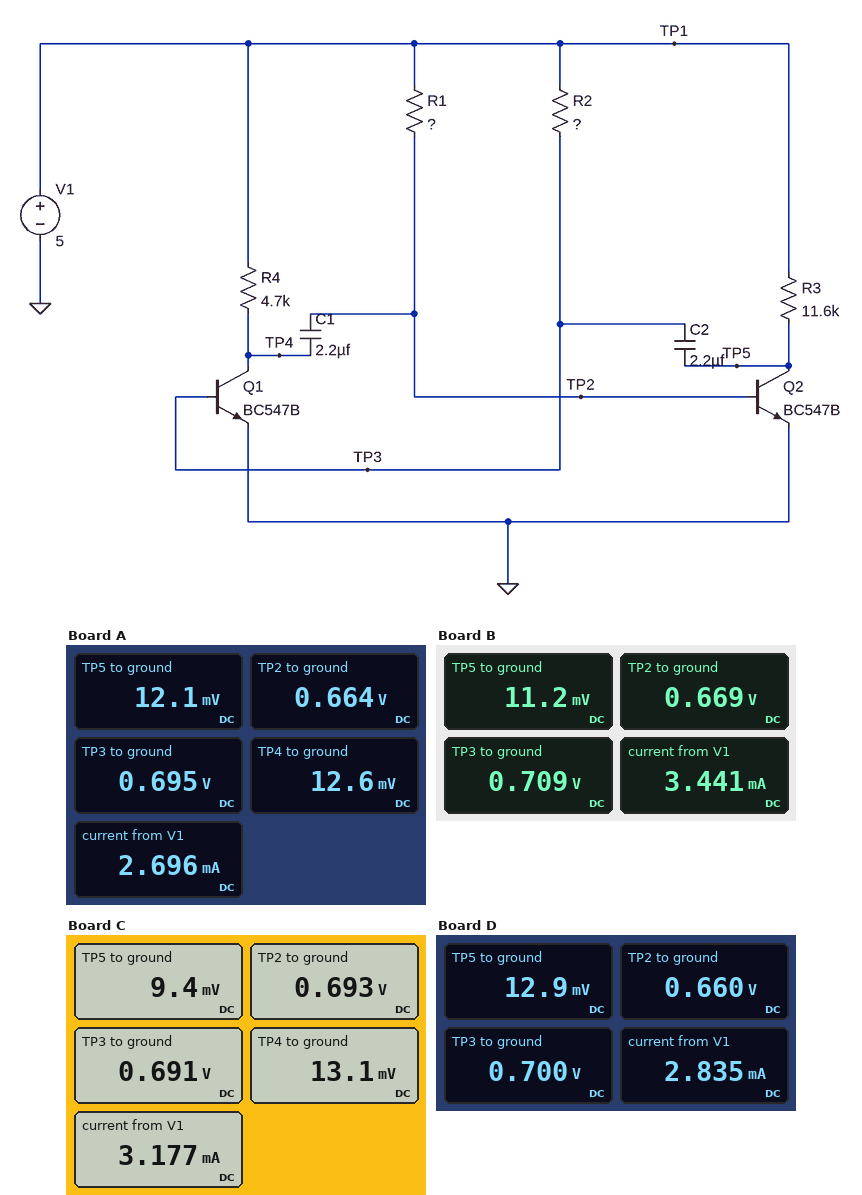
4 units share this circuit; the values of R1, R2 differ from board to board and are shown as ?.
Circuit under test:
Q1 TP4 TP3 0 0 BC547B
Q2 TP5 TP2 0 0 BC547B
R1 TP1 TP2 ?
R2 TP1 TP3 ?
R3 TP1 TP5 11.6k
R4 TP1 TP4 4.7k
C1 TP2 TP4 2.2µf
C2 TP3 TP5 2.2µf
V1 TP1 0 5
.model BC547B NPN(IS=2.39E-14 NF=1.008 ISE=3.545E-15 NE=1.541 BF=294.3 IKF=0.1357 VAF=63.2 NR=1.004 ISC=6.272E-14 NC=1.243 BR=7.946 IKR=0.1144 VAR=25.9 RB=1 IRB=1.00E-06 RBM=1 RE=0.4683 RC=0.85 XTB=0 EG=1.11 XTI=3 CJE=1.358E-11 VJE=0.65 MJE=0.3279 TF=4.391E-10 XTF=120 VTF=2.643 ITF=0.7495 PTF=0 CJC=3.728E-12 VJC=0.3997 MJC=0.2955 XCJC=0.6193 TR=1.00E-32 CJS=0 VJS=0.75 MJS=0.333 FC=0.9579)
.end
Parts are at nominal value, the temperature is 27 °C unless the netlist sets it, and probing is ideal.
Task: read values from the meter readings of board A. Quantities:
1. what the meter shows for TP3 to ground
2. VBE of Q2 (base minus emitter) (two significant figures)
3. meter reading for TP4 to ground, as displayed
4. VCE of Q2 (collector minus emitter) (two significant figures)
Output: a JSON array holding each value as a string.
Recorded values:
["0.695 V", "660 mV", "12.6 mV", "12 mV"]
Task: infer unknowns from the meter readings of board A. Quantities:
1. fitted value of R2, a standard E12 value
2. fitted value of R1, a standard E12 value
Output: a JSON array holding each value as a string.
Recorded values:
["4.7 kΩ", "15 kΩ"]
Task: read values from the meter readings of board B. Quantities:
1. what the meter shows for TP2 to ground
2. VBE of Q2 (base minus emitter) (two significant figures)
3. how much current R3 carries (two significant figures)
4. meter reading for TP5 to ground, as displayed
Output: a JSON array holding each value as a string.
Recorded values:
["0.669 V", "670 mV", "430 µA", "11.2 mV"]
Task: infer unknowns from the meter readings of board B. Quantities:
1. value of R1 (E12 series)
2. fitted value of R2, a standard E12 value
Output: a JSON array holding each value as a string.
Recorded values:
["12 kΩ", "2.7 kΩ"]
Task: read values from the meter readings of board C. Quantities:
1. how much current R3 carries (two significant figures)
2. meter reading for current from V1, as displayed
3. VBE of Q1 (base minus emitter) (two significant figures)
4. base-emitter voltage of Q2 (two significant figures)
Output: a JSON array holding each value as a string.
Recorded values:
["430 µA", "3.177 mA", "690 mV", "690 mV"]
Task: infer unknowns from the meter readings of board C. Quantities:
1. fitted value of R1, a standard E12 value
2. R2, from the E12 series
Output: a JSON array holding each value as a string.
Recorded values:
["4.7 kΩ", "5.6 kΩ"]
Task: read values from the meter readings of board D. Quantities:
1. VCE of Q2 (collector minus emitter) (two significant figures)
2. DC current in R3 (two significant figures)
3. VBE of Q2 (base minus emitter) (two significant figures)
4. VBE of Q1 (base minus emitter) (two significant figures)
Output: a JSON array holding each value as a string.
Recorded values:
["13 mV", "430 µA", "660 mV", "700 mV"]
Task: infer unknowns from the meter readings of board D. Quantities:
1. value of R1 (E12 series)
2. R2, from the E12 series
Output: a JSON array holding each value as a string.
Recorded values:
["18 kΩ", "3.9 kΩ"]
